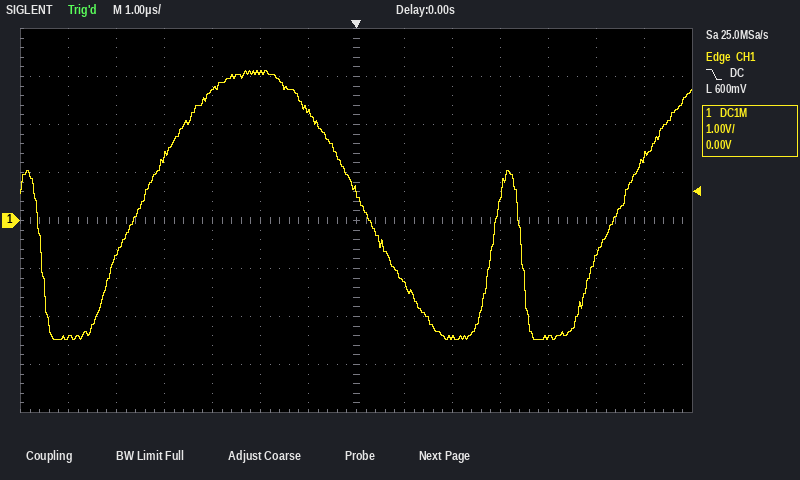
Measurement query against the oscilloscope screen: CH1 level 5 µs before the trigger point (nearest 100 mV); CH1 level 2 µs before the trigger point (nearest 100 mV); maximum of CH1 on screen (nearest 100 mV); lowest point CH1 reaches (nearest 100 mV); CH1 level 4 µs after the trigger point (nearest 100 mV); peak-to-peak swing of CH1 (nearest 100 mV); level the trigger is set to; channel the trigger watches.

-700 mV
3.1 V
3.1 V
-2.5 V
-2.4 V
5.6 V
600 mV
CH1
